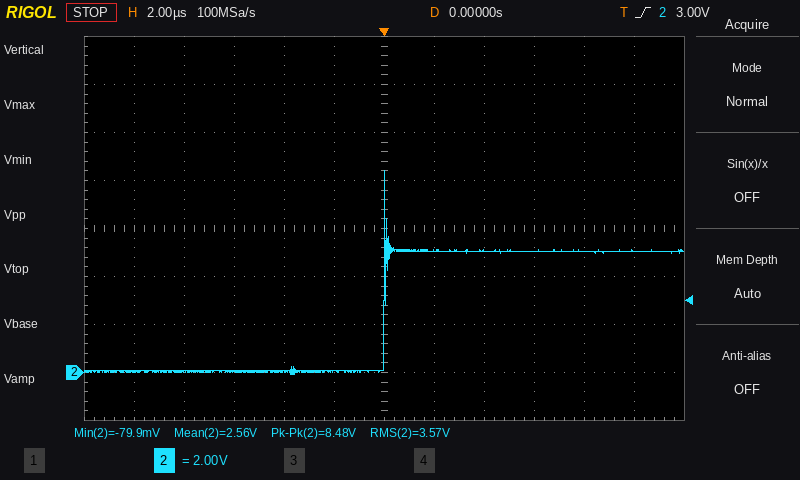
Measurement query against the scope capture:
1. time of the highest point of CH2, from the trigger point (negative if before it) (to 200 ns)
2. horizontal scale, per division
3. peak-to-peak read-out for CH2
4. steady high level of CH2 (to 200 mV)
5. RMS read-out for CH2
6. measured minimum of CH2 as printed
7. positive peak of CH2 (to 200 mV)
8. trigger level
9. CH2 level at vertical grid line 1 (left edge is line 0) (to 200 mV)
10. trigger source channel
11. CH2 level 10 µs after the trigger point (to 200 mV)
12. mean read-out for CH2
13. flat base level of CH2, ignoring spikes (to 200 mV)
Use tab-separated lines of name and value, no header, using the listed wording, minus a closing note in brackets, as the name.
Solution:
time of the highest point of CH2, from the trigger point (negative if before it)	0.0 µs
horizontal scale, per division	2 µs
peak-to-peak read-out for CH2	8.48 V
steady high level of CH2	5.0 V
RMS read-out for CH2	3.57 V
measured minimum of CH2 as printed	-79.9 mV
positive peak of CH2	8.4 V
trigger level	3.00 V
CH2 level at vertical grid line 1 (left edge is line 0)	0.0 V
trigger source channel	CH2
CH2 level 10 µs after the trigger point	5.0 V
mean read-out for CH2	2.56 V
flat base level of CH2, ignoring spikes	0.0 V
